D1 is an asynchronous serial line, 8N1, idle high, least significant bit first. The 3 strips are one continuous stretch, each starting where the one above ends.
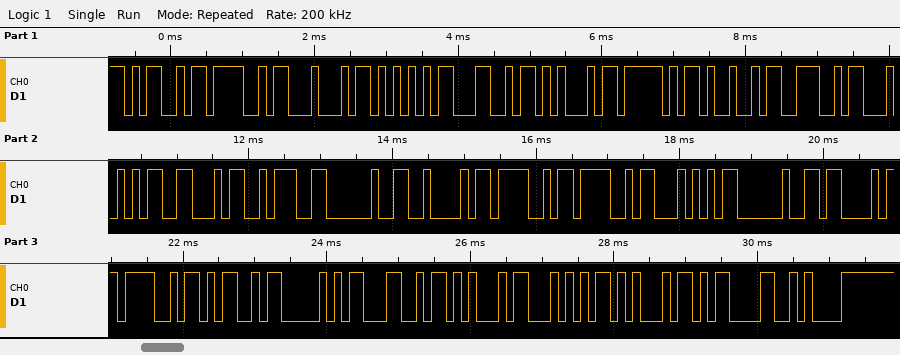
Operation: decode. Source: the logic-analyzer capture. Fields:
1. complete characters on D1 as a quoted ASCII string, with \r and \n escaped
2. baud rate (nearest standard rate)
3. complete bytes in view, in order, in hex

"MODULE_INTF: BOOT COMPLETE\r\n"
9600 baud
4D 4F 44 55 4C 45 5F 49 4E 54 46 3A 20 42 4F 4F 54 20 43 4F 4D 50 4C 45 54 45 0D 0A
